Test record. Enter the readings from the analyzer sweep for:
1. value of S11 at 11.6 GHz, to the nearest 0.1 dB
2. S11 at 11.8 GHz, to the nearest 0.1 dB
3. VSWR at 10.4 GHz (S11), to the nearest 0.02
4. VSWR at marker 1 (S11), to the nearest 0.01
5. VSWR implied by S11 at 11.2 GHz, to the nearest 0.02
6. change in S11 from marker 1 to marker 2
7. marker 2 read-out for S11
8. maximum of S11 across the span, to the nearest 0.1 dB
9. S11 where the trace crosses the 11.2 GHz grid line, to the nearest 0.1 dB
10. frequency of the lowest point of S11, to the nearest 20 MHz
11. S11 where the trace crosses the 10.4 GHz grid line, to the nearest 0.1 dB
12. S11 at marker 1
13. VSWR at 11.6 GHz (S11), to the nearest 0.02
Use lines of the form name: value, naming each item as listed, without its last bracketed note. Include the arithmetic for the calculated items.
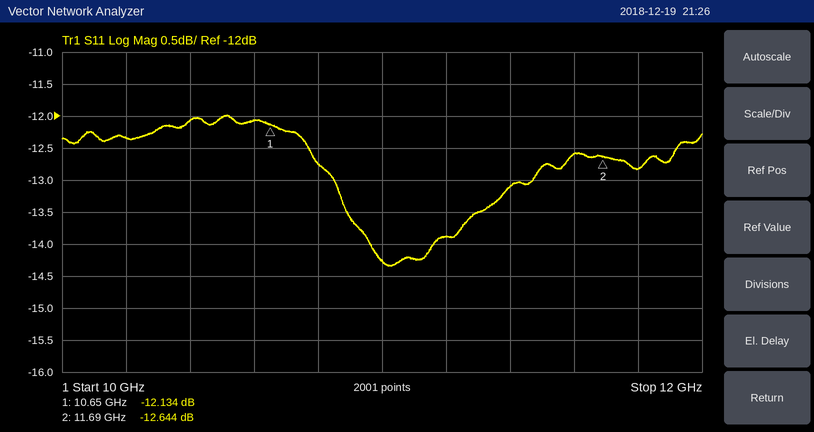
value of S11 at 11.6 GHz, to the nearest 0.1 dB: -12.6 dB
S11 at 11.8 GHz, to the nearest 0.1 dB: -12.8 dB
VSWR at 10.4 GHz (S11), to the nearest 0.02: |Γ| = 10^(-12.1/20) = 0.2483; VSWR = (1 + 0.2483)/(1 − 0.2483) ≈ 1.66
VSWR at marker 1 (S11), to the nearest 0.01: (1 + 0.2473)/(1 − 0.2473) ≈ 1.66
VSWR implied by S11 at 11.2 GHz, to the nearest 0.02: |Γ| = 10^(-13.9/20) = 0.2018; VSWR = (1 + 0.2018)/(1 − 0.2018) ≈ 1.51, so 1.50 to the nearest 0.02
change in S11 from marker 1 to marker 2: -12.644 − (-12.134) = -0.510 dB
marker 2 read-out for S11: -12.644 dB
maximum of S11 across the span, to the nearest 0.1 dB: -12.0 dB
S11 where the trace crosses the 11.2 GHz grid line, to the nearest 0.1 dB: -13.9 dB
frequency of the lowest point of S11, to the nearest 20 MHz: 11.02 GHz
S11 where the trace crosses the 10.4 GHz grid line, to the nearest 0.1 dB: -12.1 dB
S11 at marker 1: -12.134 dB
VSWR at 11.6 GHz (S11), to the nearest 0.02: |Γ| = 10^(-12.6/20) = 0.2344; VSWR = (1 + 0.2344)/(1 − 0.2344) ≈ 1.61, so 1.62 to the nearest 0.02
